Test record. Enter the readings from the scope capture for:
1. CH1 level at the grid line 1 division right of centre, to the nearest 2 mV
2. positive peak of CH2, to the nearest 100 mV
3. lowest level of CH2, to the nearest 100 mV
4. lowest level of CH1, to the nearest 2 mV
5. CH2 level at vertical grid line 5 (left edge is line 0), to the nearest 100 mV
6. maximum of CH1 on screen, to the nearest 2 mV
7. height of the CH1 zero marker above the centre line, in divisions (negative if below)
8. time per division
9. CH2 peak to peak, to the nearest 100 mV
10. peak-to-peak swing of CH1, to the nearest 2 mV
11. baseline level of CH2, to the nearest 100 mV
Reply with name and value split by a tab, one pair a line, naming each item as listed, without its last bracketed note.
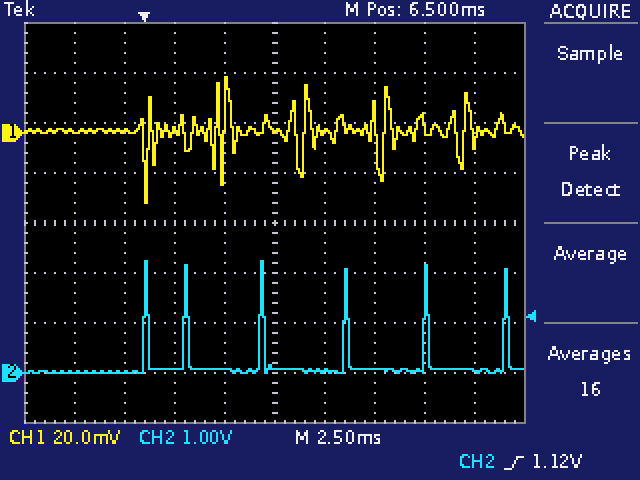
CH1 level at the grid line 1 division right of centre, to the nearest 2 mV	0 mV
positive peak of CH2, to the nearest 100 mV	2.2 V
lowest level of CH2, to the nearest 100 mV	0.0 V
lowest level of CH1, to the nearest 2 mV	-28 mV
CH2 level at vertical grid line 5 (left edge is line 0), to the nearest 100 mV	100 mV
maximum of CH1 on screen, to the nearest 2 mV	22 mV
height of the CH1 zero marker above the centre line, in divisions	+1.8 div
time per division	2.5 ms
CH2 peak to peak, to the nearest 100 mV	2.2 V
peak-to-peak swing of CH1, to the nearest 2 mV	50 mV
baseline level of CH2, to the nearest 100 mV	100 mV
